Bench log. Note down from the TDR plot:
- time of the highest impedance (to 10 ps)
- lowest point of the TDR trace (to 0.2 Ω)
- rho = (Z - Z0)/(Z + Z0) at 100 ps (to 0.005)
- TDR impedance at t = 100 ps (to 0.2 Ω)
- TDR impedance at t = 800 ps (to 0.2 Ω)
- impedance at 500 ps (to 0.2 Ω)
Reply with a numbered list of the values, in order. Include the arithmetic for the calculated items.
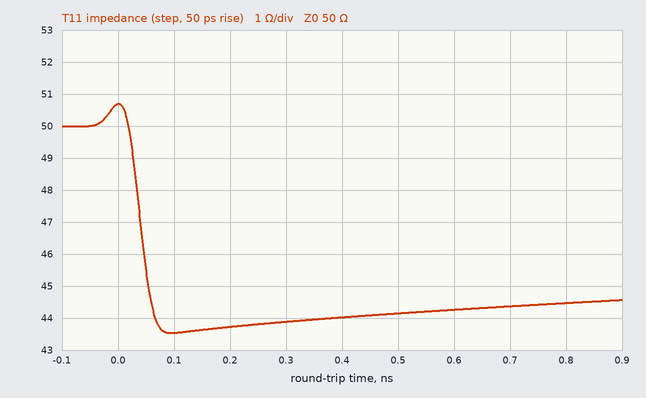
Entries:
1. 0 ps
2. 43.6 Ω
3. (43.6 − 50)/(43.6 + 50) ≈ -0.0684, so -0.070 to the nearest 0.005
4. 43.6 Ω
5. 44.4 Ω
6. 44.2 Ω
